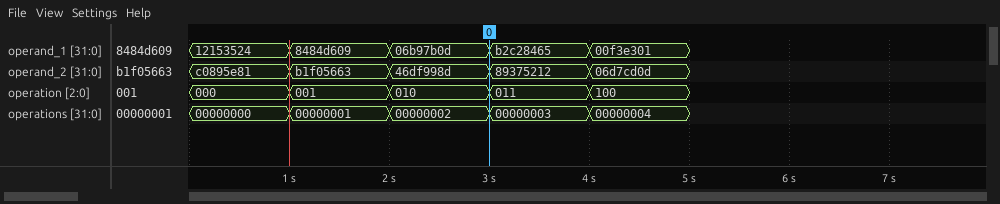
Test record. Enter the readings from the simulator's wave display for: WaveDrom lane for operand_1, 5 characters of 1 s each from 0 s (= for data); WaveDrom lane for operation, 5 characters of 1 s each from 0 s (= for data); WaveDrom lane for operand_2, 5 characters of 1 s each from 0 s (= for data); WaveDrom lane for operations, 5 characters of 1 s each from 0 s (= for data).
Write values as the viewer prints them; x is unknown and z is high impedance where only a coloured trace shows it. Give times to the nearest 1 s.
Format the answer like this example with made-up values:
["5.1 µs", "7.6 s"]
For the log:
["{name: 'operand_1', wave: '=====', data: '12153524 8484d609 06b97b0d b2c28465 00f3e301'}", "{name: 'operation', wave: '=====', data: '000 001 010 011 100'}", "{name: 'operand_2', wave: '=====', data: 'c0895e81 b1f05663 46df998d 89375212 06d7cd0d'}", "{name: 'operations', wave: '=====', data: '00000000 00000001 00000002 00000003 00000004'}"]
